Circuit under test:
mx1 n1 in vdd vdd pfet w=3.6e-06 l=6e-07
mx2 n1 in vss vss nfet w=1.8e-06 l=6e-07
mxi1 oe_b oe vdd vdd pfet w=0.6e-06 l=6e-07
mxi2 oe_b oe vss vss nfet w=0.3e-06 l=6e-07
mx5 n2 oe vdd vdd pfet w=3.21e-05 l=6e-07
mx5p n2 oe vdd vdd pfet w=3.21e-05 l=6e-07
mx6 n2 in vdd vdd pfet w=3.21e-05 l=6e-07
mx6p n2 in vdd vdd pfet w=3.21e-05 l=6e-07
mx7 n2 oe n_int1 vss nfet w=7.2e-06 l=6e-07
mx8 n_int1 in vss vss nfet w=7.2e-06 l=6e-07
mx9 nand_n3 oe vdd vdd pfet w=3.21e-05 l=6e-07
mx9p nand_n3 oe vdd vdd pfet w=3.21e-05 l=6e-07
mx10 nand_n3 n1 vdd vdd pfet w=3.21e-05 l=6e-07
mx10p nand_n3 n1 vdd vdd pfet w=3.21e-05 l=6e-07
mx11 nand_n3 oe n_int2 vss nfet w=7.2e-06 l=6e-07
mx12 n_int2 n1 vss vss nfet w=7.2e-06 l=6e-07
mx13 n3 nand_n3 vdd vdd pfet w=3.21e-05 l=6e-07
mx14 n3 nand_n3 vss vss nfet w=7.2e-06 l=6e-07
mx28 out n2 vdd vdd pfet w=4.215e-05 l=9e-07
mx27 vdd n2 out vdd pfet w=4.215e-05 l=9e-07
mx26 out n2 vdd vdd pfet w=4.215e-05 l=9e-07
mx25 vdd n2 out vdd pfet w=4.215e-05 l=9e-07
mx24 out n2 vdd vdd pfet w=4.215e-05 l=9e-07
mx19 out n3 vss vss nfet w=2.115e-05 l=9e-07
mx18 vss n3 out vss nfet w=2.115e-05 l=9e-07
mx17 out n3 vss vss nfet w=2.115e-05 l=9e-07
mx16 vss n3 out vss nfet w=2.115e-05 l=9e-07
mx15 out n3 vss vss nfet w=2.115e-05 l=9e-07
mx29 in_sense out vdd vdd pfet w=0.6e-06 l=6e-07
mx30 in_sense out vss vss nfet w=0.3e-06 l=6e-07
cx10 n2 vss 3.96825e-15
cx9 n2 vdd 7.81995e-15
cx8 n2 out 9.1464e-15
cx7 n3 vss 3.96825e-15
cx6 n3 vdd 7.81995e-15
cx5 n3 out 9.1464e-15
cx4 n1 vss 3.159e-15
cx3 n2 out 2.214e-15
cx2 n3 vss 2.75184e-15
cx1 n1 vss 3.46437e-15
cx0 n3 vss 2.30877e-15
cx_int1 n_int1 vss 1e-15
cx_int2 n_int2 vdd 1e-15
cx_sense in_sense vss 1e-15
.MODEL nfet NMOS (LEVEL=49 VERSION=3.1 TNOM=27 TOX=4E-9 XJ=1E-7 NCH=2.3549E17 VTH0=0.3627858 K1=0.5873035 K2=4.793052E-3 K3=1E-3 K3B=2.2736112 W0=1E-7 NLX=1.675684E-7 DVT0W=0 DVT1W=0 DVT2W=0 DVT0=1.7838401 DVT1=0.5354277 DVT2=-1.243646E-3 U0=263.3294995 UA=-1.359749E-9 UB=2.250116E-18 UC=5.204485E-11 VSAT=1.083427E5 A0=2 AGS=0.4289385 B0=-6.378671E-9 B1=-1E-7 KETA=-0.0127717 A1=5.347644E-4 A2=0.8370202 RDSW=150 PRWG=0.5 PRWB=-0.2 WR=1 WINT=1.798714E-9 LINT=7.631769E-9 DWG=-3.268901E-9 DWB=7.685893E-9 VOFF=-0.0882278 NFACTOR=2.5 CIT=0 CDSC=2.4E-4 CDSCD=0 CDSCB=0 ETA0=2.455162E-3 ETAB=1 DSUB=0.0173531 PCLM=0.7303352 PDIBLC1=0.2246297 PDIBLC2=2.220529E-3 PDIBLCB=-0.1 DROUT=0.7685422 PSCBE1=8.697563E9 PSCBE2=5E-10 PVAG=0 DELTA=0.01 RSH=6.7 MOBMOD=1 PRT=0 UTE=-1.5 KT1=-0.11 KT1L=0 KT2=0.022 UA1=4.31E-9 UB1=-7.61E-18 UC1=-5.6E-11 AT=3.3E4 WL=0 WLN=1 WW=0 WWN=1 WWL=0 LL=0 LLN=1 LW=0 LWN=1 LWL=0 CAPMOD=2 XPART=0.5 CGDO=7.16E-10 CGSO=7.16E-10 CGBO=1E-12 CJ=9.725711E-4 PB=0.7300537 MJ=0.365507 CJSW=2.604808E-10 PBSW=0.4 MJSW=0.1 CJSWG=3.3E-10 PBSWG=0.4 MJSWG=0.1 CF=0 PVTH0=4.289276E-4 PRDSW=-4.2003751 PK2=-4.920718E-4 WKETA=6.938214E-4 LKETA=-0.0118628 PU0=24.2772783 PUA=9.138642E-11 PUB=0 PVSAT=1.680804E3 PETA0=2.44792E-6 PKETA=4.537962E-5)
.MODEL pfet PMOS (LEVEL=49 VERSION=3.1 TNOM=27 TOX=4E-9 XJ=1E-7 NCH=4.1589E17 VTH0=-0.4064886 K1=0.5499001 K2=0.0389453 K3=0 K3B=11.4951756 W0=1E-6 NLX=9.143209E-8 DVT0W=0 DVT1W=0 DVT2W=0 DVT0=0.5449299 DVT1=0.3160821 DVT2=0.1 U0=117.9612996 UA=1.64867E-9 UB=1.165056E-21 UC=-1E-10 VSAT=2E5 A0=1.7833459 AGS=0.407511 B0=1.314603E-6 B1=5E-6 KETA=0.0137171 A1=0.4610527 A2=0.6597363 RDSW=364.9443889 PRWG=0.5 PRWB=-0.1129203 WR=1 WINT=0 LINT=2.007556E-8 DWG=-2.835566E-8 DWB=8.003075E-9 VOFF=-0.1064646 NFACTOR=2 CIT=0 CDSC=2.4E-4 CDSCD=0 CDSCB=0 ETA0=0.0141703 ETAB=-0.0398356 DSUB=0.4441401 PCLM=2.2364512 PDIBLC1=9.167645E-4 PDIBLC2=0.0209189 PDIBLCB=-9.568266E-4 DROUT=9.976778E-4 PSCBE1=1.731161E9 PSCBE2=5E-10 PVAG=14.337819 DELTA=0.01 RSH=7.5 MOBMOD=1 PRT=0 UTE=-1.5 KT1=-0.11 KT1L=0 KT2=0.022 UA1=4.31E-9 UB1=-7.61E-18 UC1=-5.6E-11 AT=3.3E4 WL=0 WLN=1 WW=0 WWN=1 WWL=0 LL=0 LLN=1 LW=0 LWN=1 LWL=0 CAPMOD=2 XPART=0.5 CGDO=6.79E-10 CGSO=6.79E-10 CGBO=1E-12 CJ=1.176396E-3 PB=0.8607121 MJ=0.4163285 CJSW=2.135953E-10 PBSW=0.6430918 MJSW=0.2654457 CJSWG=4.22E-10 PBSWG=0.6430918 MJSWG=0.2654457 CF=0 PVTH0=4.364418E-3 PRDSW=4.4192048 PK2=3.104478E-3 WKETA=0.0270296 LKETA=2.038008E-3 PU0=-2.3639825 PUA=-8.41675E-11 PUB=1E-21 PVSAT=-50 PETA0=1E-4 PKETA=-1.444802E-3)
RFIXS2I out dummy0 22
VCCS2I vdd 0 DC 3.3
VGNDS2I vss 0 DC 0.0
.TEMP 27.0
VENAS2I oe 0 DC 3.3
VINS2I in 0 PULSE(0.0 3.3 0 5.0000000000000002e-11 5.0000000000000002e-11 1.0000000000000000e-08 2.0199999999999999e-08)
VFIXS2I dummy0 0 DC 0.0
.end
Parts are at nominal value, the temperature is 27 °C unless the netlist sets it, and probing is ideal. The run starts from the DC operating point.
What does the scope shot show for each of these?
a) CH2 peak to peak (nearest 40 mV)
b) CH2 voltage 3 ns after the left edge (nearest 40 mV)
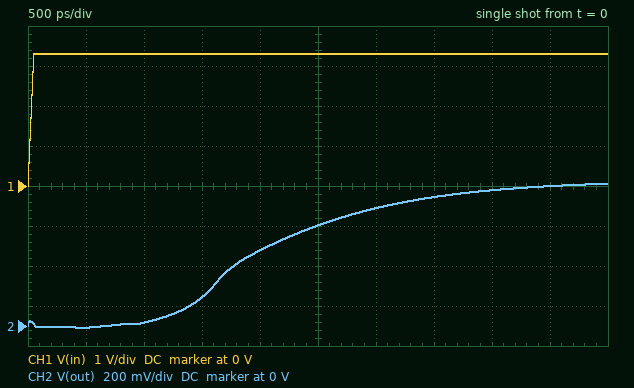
720 mV
600 mV
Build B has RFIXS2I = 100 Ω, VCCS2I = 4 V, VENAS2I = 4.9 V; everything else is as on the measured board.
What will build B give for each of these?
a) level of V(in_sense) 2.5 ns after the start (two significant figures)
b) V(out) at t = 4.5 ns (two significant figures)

190 mV
2.7 V
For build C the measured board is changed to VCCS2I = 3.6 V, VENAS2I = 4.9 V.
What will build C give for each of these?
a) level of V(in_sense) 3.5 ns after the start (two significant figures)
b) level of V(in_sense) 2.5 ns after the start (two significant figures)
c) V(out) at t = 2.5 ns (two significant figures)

3.5 V
3.6 V
630 mV
